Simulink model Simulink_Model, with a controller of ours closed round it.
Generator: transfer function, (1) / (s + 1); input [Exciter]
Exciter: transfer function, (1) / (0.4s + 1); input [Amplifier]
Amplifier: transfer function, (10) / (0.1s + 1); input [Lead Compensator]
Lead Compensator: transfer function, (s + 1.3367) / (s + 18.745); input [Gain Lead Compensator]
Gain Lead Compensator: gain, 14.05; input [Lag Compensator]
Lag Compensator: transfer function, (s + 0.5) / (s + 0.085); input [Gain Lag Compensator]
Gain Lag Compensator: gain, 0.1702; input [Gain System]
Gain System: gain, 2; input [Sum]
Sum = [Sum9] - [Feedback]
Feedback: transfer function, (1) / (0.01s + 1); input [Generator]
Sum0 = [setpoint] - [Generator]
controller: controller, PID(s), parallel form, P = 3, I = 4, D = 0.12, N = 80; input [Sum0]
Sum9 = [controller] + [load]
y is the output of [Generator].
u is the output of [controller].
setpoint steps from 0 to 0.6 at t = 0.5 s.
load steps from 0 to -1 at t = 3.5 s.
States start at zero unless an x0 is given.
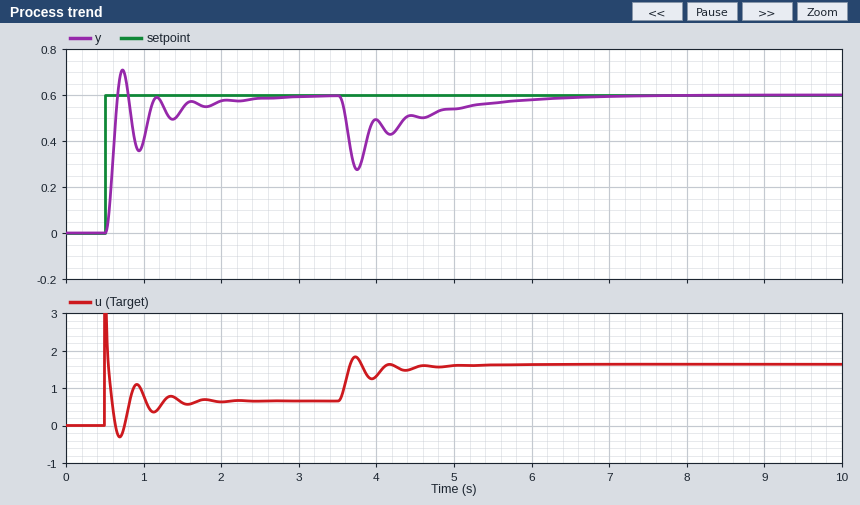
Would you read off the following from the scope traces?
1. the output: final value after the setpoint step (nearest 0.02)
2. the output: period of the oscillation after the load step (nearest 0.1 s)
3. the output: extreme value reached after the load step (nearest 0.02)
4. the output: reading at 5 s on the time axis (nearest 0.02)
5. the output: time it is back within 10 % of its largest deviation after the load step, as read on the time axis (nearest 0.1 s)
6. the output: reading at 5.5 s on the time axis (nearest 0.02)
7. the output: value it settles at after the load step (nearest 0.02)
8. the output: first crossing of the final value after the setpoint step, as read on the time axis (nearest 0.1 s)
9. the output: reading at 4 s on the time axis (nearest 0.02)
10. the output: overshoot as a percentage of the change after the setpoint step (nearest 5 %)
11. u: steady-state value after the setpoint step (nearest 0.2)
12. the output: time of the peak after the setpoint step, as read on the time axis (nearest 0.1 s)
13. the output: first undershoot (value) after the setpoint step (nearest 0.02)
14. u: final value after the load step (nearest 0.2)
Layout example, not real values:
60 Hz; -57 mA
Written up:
0.60; 0.4 s; 0.28; 0.54; 5.6 s; 0.56; 0.60; 0.7 s; 0.50; 20 %; 0.6; 0.7 s; 0.36; 1.6
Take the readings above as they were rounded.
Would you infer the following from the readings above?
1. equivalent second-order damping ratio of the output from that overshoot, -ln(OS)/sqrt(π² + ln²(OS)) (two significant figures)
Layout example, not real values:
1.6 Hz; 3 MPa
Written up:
0.46
